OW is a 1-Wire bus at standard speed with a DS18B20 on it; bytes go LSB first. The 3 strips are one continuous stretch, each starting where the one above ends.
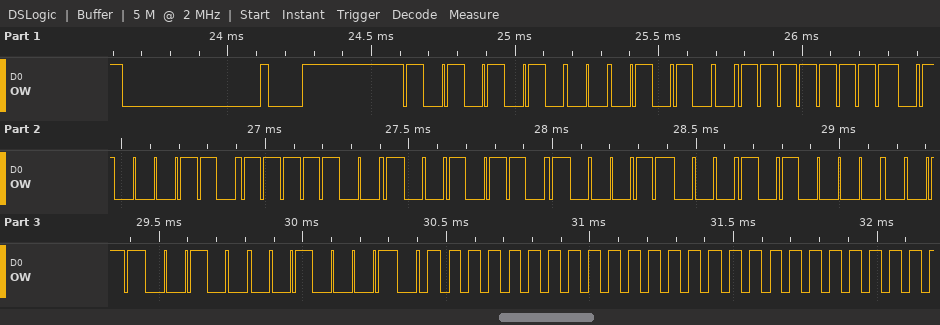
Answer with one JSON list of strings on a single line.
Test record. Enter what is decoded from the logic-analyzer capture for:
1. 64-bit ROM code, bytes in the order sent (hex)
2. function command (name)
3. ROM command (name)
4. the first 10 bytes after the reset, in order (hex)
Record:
["28 FF 62 9F B4 18 05 26", "Convert T", "Match ROM", "55 28 FF 62 9F B4 18 05 26 44"]
